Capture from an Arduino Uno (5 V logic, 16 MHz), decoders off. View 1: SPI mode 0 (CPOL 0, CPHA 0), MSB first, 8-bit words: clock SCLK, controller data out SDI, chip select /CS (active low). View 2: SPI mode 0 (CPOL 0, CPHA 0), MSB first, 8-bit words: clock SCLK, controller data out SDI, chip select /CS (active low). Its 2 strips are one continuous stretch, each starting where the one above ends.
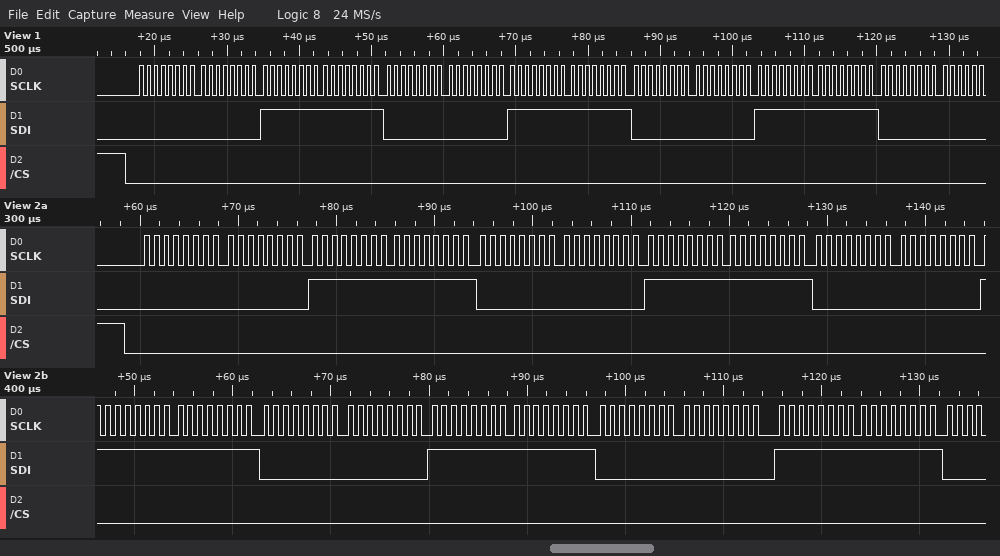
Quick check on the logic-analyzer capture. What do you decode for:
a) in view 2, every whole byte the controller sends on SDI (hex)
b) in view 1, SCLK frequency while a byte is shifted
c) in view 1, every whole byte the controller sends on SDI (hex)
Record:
00 00 FF FF 00 00 FF FF 00 00 FF FF 00 00 FF FF 00 00 FF FF
1 MHz
0x00 0x00 0xFF 0xFF 0x00 0x00 0xFF 0xFF 0x00 0x00 0xFF 0xFF 0x00
